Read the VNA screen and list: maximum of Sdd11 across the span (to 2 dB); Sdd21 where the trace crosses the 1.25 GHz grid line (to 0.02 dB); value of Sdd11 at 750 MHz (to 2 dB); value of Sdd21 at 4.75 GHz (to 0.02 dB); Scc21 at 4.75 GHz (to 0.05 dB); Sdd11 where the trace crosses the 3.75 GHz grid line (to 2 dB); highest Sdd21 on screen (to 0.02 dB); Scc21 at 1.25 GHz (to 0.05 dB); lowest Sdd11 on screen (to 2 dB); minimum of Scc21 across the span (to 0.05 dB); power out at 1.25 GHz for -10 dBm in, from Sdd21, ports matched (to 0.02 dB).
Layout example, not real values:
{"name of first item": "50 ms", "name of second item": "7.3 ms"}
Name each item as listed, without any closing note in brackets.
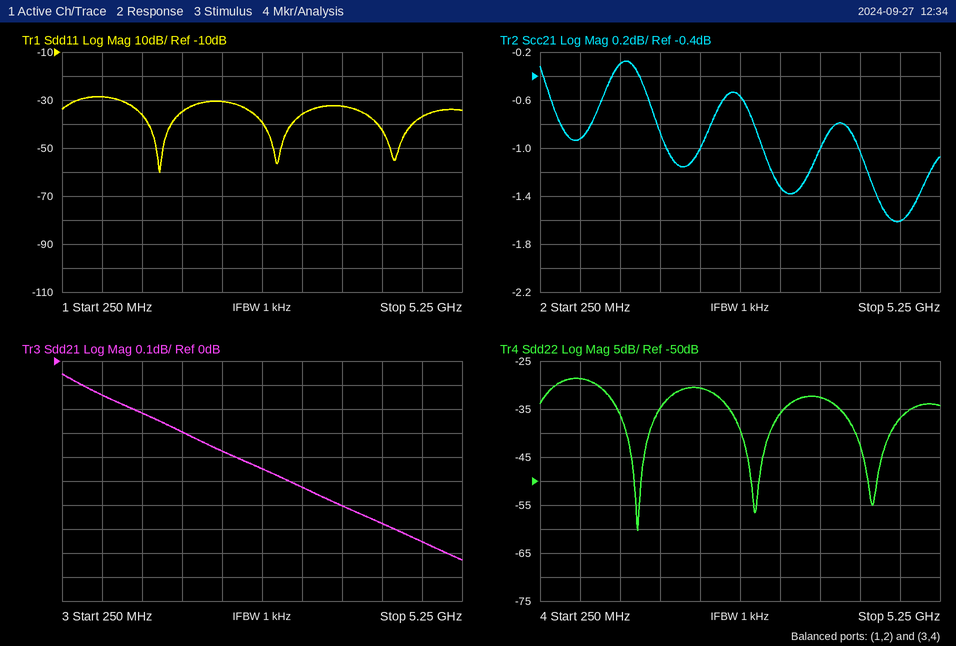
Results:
{"maximum of Sdd11 across the span": "-28 dB", "Sdd21 where the trace crosses the 1.25 GHz grid line": "-0.22 dB", "value of Sdd11 at 750 MHz": "-28 dB", "value of Sdd21 at 4.75 GHz": "-0.76 dB", "Scc21 at 4.75 GHz": "-1.60 dB", "Sdd11 where the trace crosses the 3.75 GHz grid line": "-32 dB", "highest Sdd21 on screen": "-0.06 dB", "Scc21 at 1.25 GHz": "-0.30 dB", "lowest Sdd11 on screen": "-60 dB", "minimum of Scc21 across the span": "-1.60 dB", "power out at 1.25 GHz for -10 dBm in, from Sdd21, ports matched": "-10.22 dBm"}
